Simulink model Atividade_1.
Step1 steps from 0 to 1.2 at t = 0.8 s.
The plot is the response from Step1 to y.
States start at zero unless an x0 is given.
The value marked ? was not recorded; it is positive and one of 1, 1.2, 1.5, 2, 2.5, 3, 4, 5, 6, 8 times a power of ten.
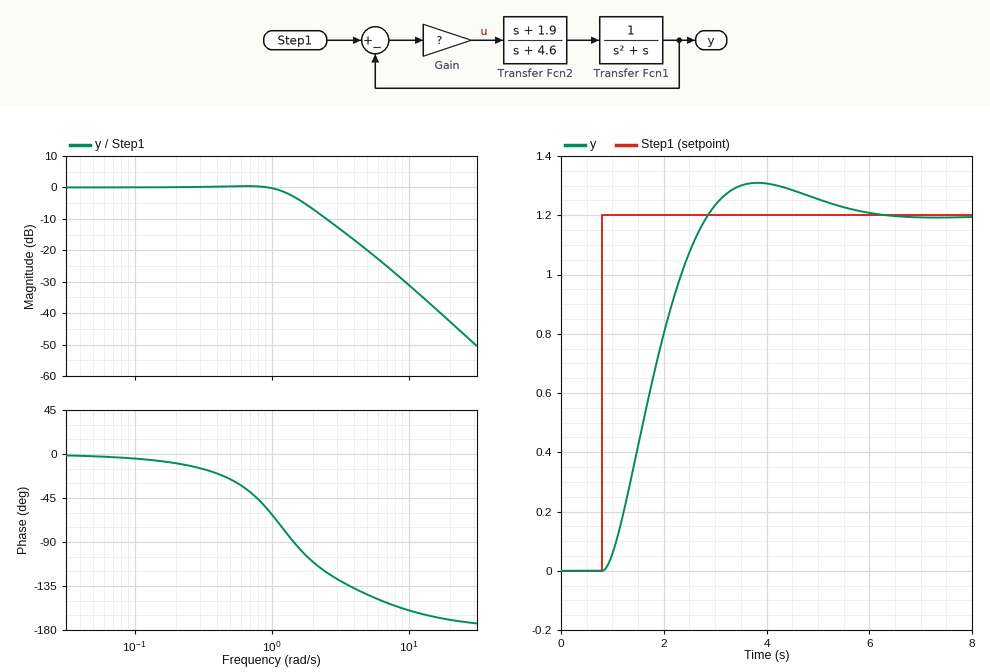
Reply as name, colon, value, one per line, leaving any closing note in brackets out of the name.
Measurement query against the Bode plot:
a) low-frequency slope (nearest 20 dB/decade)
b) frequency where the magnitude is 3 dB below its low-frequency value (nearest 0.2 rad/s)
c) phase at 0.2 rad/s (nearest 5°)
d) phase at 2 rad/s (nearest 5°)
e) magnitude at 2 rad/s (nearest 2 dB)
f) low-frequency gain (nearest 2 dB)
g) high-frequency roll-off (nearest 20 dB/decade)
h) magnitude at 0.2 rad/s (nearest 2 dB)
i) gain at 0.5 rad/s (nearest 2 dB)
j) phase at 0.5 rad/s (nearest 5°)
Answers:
low-frequency slope: 0 dB/decade
frequency where the magnitude is 3 dB below its low-frequency value: 1.4 rad/s
phase at 0.2 rad/s: -10°
phase at 2 rad/s: -110°
magnitude at 2 rad/s: -6 dB
low-frequency gain: 0 dB
high-frequency roll-off: -40 dB/decade
magnitude at 0.2 rad/s: 0 dB
gain at 0.5 rad/s: 0 dB
phase at 0.5 rad/s: -25°
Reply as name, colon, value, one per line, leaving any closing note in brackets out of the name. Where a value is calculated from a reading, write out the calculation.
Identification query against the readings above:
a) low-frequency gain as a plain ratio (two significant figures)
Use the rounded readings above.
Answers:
low-frequency gain as a plain ratio: 10^(0 / 20) = 1.0
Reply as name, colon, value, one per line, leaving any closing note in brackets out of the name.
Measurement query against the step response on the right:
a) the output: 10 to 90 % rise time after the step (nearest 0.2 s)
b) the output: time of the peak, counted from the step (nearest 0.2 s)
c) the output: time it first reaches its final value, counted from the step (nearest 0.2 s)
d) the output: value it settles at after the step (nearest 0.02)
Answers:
the output: 10 to 90 % rise time after the step: 1.4 s
the output: time of the peak, counted from the step: 3.0 s
the output: time it first reaches its final value, counted from the step: 2.0 s
the output: value it settles at after the step: 1.20
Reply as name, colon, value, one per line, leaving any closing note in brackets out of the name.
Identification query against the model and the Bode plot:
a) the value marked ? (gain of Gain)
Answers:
the value marked ?: 3
